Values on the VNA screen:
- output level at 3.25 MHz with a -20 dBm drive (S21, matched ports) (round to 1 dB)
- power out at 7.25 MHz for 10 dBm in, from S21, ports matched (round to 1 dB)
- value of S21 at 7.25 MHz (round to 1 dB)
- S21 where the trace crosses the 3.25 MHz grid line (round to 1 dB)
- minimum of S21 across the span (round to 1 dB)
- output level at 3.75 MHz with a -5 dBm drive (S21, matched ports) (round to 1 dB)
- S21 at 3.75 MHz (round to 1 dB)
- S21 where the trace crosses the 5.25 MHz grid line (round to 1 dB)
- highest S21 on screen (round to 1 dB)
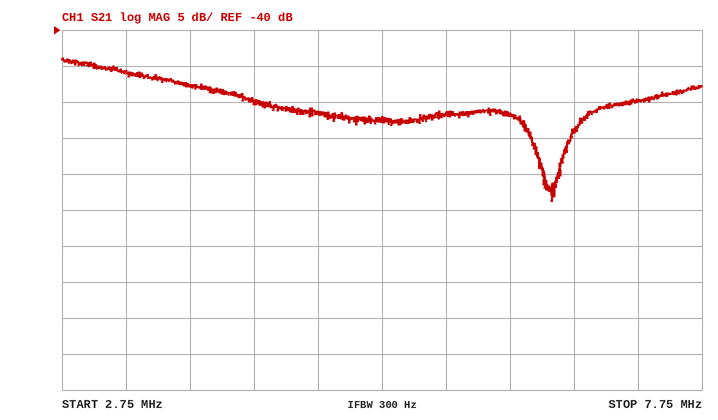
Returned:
-66 dBm
-40 dBm
-50 dB
-46 dB
-64 dB
-53 dBm
-48 dB
-52 dB
-44 dB
